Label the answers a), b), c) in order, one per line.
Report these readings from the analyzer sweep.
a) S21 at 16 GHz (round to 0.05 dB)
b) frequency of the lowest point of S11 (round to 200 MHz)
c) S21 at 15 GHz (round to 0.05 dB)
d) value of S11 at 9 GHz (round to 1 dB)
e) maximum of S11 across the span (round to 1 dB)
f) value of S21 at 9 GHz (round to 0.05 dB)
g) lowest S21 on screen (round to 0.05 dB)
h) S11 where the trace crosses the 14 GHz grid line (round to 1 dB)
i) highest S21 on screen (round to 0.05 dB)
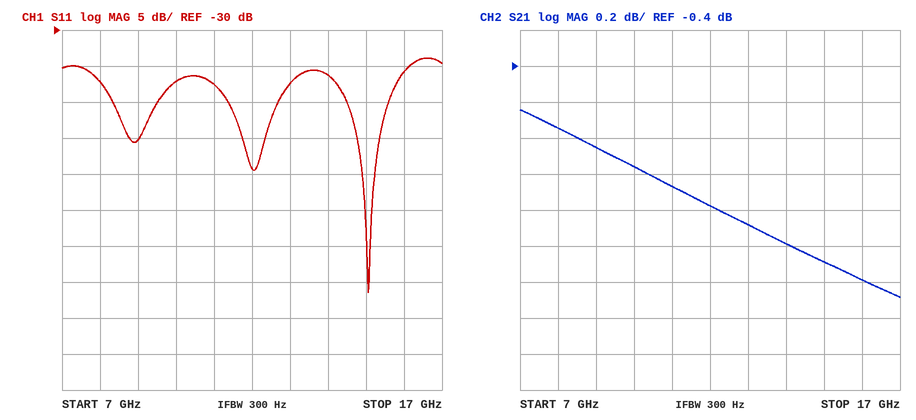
a) -1.60 dB
b) 15.0 GHz
c) -1.50 dB
d) -45 dB
e) -34 dB
f) -0.85 dB
g) -1.70 dB
h) -36 dB
i) -0.65 dB
